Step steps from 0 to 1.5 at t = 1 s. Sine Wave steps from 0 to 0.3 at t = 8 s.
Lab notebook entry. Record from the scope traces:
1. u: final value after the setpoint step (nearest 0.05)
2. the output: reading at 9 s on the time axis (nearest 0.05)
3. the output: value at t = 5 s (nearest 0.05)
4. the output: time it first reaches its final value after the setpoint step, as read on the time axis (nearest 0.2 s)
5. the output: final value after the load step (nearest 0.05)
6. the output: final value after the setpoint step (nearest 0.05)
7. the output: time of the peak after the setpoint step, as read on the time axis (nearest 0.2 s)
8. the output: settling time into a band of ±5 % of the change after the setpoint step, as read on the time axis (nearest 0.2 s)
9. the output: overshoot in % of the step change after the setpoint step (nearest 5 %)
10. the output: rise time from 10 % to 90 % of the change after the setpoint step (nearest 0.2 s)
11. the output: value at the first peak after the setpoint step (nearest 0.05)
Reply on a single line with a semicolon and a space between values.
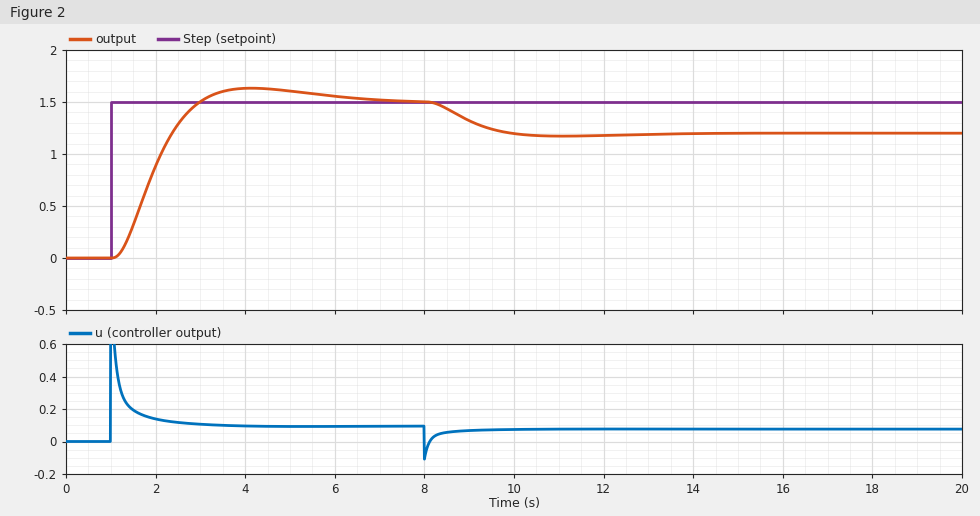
0.10; 1.30; 1.60; 3.0 s; 1.20; 1.50; 4.2 s; 5.6 s; 10 %; 1.2 s; 1.65
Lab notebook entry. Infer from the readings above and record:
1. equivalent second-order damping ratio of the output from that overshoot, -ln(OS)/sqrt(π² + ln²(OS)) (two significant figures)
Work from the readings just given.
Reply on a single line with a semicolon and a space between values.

0.59
